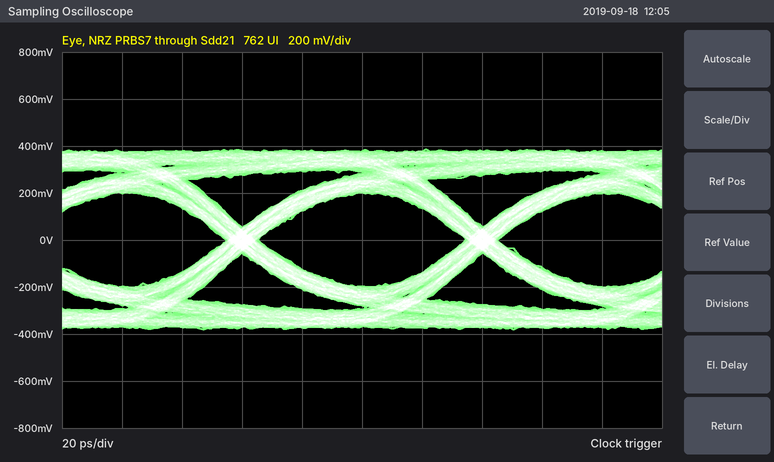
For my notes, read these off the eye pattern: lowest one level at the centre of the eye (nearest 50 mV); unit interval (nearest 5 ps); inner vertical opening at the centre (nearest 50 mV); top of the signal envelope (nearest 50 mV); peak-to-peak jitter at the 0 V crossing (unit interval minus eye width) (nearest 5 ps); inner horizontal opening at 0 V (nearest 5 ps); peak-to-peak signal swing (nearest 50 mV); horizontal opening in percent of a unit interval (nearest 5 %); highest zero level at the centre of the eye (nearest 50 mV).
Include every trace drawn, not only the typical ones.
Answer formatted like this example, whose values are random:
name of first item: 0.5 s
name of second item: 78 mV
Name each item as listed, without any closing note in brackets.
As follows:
lowest one level at the centre of the eye: 200 mV
unit interval: 80 ps
inner vertical opening at the centre: 400 mV
top of the signal envelope: 400 mV
peak-to-peak jitter at the 0 V crossing (unit interval minus eye width): 10 ps
inner horizontal opening at 0 V: 70 ps
peak-to-peak signal swing: 750 mV
horizontal opening in percent of a unit interval: 85 %
highest zero level at the centre of the eye: -200 mV
